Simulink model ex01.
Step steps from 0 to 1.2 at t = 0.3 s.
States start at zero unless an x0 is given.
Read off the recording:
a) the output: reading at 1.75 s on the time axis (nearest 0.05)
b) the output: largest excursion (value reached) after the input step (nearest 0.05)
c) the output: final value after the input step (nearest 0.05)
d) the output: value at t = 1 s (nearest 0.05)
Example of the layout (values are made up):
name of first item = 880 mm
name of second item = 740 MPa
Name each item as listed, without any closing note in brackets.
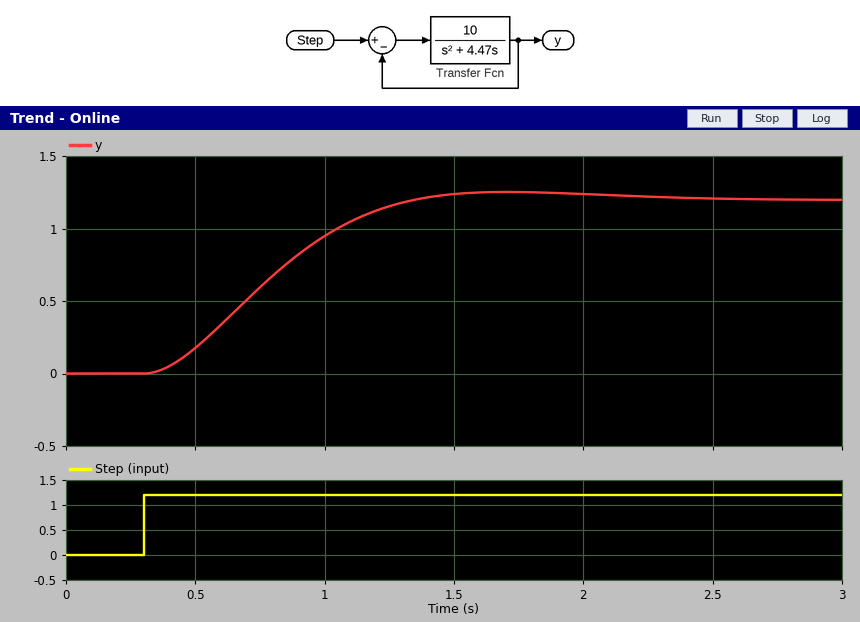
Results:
the output: reading at 1.75 s on the time axis = 1.25
the output: largest excursion (value reached) after the input step = 1.25
the output: final value after the input step = 1.20
the output: value at t = 1 s = 0.95
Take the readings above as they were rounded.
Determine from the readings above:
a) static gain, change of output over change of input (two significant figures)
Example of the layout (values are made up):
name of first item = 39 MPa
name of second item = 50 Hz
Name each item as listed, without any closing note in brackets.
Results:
static gain, change of output over change of input = 1.0
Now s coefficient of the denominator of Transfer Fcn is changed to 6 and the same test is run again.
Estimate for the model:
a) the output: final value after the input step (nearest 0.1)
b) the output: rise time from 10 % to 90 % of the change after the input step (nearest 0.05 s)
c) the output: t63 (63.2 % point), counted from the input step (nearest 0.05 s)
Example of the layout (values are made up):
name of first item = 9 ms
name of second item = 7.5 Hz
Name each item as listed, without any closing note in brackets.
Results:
the output: final value after the input step = 1.2
the output: rise time from 10 % to 90 % of the change after the input step = 1.00 s
the output: t63 (63.2 % point), counted from the input step = 0.65 s
